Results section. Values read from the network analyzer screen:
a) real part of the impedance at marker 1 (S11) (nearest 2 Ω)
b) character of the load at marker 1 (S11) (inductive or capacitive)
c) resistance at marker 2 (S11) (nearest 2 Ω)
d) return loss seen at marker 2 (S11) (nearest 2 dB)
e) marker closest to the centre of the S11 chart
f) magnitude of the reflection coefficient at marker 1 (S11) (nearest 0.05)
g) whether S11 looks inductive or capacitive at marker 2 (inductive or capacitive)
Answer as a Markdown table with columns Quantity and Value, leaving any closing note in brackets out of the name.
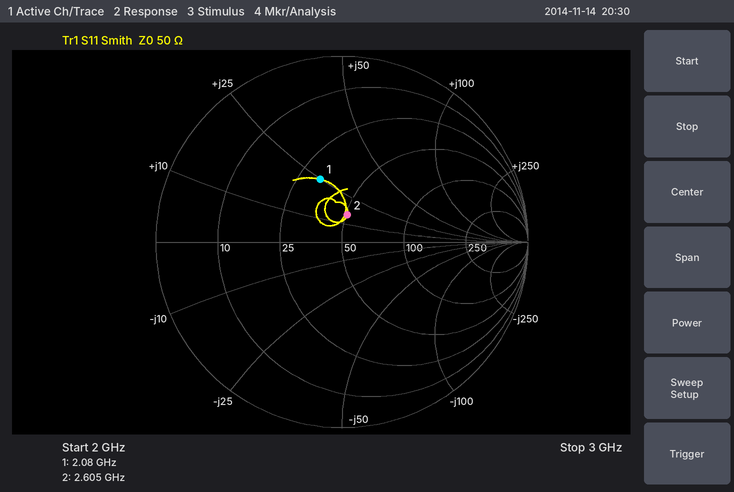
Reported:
| Quantity | Value |
|---|---|
| real part of the impedance at marker 1 (S11) | 32 Ω |
| character of the load at marker 1 (S11) | inductive |
| resistance at marker 2 (S11) | 50 Ω |
| return loss seen at marker 2 (S11) | 16 dB |
| marker closest to the centre of the S11 chart | marker 2 |
| magnitude of the reflection coefficient at marker 1 (S11) | 0.35 |
| whether S11 looks inductive or capacitive at marker 2 | inductive |
